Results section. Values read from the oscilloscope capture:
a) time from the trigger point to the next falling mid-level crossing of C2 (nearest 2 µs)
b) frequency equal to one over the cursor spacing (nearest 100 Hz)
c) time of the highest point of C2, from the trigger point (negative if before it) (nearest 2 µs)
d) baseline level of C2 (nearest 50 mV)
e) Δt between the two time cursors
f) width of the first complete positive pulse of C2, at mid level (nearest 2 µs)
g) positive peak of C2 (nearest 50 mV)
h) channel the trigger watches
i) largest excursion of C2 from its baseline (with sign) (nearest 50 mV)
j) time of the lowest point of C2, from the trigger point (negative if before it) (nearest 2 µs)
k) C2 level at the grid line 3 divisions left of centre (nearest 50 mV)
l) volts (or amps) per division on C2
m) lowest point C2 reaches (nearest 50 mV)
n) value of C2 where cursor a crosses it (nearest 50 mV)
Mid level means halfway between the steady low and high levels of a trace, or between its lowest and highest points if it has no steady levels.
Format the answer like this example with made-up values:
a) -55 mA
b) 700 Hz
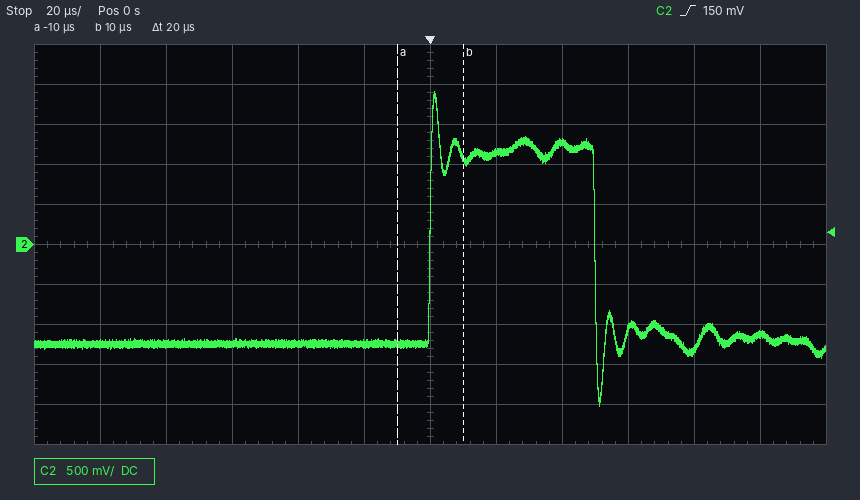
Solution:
a) 50 µs
b) 50.0 kHz
c) +2 µs
d) -1.25 V
e) 20 µs
f) 50 µs
g) 1.90 V
h) C2
i) +3.15 V
j) +52 µs
k) -1.25 V
l) 500 mV
m) -2.00 V
n) -1.25 V
